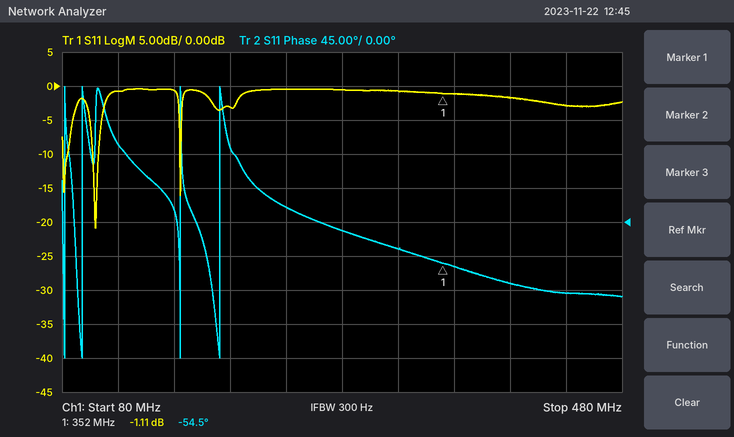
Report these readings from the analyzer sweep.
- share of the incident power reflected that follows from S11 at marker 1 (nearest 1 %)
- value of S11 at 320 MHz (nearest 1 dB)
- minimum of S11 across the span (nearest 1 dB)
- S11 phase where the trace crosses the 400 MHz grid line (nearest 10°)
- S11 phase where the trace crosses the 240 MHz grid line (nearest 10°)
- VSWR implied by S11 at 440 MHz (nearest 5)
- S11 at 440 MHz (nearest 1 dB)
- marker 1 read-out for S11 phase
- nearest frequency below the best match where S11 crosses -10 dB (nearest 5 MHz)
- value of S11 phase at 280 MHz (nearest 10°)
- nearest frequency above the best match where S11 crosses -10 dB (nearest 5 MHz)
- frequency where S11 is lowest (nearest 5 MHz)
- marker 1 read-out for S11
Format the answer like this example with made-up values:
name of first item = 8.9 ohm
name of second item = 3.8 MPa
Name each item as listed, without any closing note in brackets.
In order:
share of the incident power reflected that follows from S11 at marker 1 = 77 %
value of S11 at 320 MHz = -1 dB
minimum of S11 across the span = -21 dB
S11 phase where the trace crosses the 400 MHz grid line = -80°
S11 phase where the trace crosses the 240 MHz grid line = 20°
VSWR implied by S11 at 440 MHz = 5
S11 at 440 MHz = -3 dB
marker 1 read-out for S11 phase = -54.5°
nearest frequency below the best match where S11 crosses -10 dB = 100 MHz
value of S11 phase at 280 MHz = -10°
nearest frequency above the best match where S11 crosses -10 dB = 105 MHz
frequency where S11 is lowest = 105 MHz
marker 1 read-out for S11 = -1.11 dB
